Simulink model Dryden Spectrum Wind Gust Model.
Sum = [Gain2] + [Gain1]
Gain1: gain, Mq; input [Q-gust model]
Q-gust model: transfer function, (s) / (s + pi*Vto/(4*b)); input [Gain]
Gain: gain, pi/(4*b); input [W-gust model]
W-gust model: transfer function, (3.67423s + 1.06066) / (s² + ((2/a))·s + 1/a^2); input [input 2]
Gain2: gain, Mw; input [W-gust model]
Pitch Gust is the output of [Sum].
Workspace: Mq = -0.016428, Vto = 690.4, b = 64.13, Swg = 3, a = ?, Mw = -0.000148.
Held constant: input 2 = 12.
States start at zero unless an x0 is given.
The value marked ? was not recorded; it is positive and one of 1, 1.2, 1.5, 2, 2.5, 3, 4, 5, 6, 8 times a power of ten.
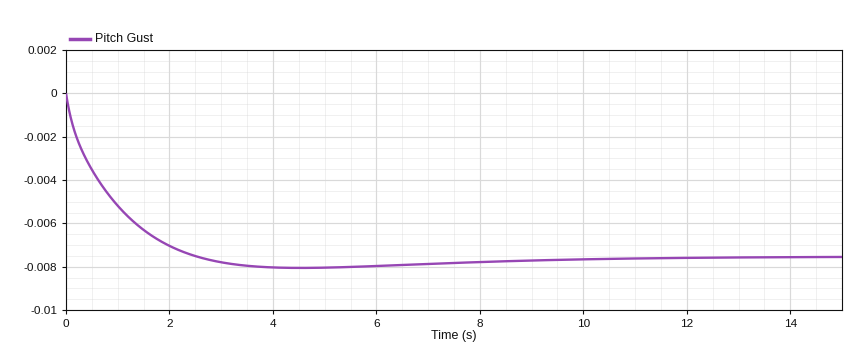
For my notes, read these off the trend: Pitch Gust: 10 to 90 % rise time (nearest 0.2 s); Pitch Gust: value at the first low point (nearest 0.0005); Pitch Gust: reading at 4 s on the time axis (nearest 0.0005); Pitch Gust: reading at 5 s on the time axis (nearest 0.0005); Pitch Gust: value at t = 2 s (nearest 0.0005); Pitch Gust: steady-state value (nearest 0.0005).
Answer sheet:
1.8 s
-0.0080
-0.0080
-0.0080
-0.0070
-0.0075
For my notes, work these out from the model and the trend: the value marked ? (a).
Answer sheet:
2
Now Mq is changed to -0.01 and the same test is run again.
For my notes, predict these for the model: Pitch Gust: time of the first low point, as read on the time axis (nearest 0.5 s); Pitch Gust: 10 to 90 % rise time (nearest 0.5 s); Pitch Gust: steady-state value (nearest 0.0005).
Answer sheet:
4.5 s
2.0 s
-0.0075
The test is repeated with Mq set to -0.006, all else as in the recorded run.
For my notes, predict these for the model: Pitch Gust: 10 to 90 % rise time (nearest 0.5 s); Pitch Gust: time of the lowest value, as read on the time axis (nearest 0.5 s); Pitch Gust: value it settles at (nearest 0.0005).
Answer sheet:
2.0 s
4.5 s
-0.0075
